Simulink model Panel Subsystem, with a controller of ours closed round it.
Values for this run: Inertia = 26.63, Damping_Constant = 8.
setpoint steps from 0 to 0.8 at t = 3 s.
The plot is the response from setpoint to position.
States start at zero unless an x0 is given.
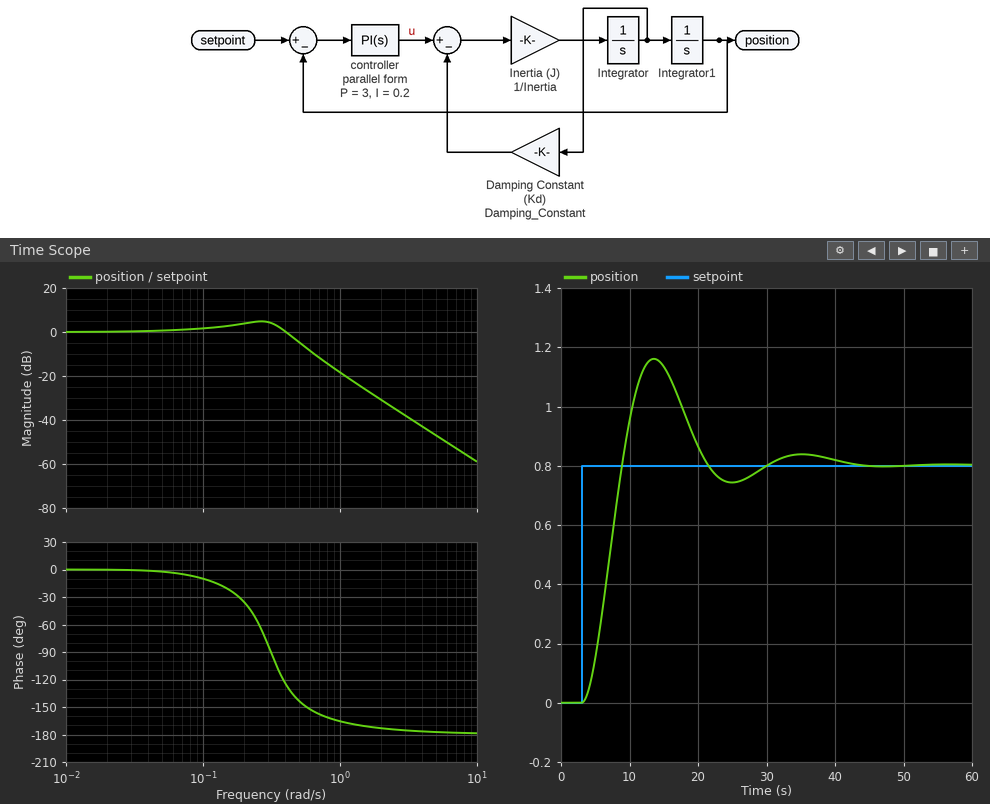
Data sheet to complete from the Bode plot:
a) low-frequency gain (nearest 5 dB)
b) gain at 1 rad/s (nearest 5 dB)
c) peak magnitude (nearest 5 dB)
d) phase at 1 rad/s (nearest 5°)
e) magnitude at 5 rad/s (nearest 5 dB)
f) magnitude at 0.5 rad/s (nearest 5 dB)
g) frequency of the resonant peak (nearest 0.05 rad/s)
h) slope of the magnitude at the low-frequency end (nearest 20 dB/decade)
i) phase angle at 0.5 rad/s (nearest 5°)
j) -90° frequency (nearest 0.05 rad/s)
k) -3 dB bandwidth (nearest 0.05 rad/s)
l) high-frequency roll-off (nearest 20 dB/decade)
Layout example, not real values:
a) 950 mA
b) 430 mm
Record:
a) 0 dB
b) -20 dB
c) 5 dB
d) -165°
e) -45 dB
f) -5 dB
g) 0.25 rad/s
h) 0 dB/decade
i) -145°
j) 0.30 rad/s
k) 0.45 rad/s
l) -40 dB/decade
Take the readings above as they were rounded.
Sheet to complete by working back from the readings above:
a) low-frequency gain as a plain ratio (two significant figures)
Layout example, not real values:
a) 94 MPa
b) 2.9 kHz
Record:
a) 1.0
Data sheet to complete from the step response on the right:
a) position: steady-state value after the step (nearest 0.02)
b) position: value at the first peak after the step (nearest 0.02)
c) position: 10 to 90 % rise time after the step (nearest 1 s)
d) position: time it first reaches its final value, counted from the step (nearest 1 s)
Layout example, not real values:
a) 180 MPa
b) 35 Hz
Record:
a) 0.80
b) 1.16
c) 4 s
d) 6 s
